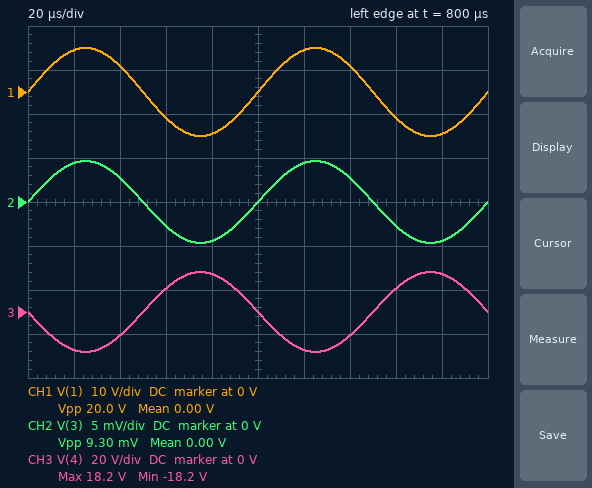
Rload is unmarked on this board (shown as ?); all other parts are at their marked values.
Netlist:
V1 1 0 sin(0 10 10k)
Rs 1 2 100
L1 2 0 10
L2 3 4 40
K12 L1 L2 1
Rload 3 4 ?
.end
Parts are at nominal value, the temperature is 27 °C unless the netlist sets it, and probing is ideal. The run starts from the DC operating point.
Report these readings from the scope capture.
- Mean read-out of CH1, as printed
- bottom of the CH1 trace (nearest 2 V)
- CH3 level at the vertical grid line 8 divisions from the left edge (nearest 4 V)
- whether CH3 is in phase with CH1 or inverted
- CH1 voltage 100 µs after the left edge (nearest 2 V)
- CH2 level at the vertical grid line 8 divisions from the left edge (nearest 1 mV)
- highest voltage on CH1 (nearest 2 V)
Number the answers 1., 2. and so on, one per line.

1. 0.00 V
2. -10 V
3. 12 V
4. inverted
5. 0 V
6. -3 mV
7. 10 V
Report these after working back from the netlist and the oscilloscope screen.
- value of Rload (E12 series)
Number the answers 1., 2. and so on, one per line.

1. 3.9 kΩ
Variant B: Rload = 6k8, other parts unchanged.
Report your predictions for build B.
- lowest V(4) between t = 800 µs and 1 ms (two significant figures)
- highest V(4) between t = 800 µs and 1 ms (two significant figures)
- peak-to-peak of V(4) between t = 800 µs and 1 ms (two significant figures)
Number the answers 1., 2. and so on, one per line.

1. -19 V
2. 19 V
3. 38 V
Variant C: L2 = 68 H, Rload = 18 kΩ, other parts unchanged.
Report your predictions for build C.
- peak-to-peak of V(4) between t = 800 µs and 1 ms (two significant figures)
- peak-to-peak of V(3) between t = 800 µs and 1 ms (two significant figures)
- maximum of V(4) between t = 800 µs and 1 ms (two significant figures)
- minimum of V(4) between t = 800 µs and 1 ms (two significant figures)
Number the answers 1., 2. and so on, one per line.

1. 50 V
2. 2.8 mV
3. 25 V
4. -25 V
